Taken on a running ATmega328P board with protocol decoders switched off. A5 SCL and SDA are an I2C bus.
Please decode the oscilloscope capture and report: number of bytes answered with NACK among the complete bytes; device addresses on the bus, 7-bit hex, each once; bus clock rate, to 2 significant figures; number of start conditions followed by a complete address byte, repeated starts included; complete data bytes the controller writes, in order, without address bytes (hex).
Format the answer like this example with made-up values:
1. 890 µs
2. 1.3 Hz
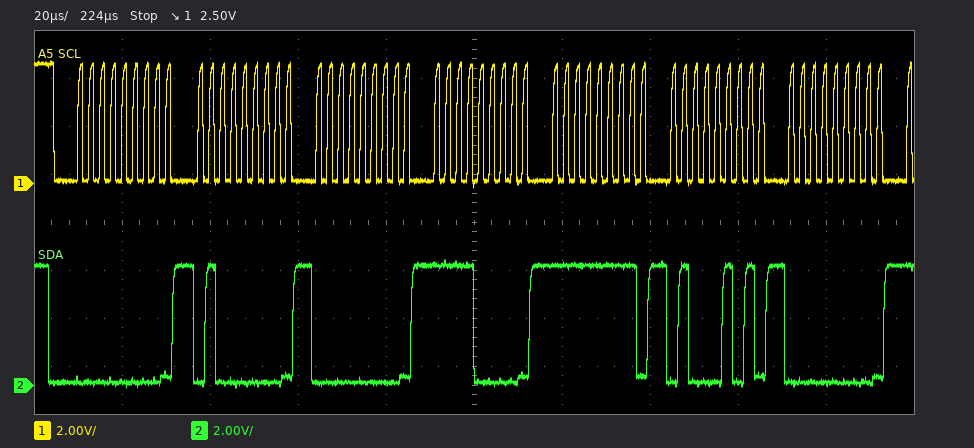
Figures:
1. 0
2. 0x00
3. 400 kHz
4. 1
5. 40 00 F0 FF 45 00
